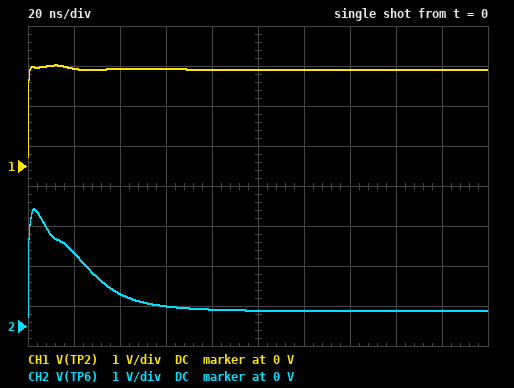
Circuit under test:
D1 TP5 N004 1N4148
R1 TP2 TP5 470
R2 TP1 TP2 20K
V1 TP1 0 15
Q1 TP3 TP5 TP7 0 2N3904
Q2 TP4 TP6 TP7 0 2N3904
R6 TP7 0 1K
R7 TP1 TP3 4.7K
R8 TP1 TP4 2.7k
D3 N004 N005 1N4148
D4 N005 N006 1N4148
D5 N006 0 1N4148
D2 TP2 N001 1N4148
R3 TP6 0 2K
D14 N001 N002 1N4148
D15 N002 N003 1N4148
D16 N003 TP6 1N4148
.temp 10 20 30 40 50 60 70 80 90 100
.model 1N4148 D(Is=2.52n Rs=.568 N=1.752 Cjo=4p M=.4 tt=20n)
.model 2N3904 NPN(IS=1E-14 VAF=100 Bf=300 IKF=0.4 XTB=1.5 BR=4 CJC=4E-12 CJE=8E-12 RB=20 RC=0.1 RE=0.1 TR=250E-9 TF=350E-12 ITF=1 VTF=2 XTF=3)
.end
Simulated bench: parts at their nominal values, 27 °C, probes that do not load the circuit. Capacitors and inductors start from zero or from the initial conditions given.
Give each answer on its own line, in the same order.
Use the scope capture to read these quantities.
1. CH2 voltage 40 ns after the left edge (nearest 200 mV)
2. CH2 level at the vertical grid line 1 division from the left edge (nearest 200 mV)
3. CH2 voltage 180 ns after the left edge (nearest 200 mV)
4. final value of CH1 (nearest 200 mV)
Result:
800 mV
1.8 V
400 mV
2.4 V
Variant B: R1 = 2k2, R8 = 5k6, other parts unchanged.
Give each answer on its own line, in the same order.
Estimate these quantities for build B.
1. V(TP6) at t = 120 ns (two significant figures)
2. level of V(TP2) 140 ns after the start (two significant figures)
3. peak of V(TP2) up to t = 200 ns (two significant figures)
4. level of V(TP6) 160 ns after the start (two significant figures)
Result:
640 mV
2.8 V
3.4 V
630 mV
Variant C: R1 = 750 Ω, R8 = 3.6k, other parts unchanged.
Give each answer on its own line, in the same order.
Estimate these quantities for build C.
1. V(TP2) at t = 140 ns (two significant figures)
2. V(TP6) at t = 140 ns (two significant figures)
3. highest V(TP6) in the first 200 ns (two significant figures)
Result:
2.5 V
430 mV
2.7 V
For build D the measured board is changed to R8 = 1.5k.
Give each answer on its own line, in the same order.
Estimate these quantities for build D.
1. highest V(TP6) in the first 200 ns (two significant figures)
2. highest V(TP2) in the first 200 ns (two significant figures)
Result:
3.5 V
2.7 V
